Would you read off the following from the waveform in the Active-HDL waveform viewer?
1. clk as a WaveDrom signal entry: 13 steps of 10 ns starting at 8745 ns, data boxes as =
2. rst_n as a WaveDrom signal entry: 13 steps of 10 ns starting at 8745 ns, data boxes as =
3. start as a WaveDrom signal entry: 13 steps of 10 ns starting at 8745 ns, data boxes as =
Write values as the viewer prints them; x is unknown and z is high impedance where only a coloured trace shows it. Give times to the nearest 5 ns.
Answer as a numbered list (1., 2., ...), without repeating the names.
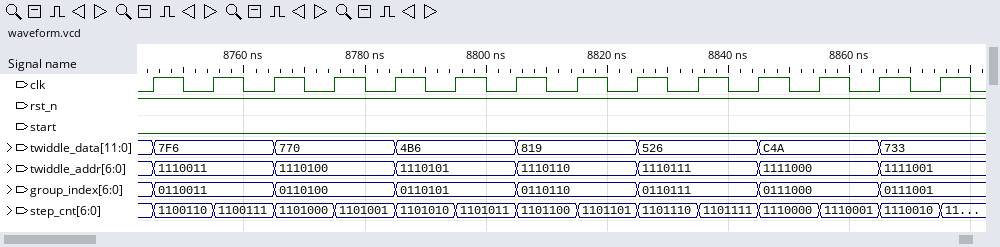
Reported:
1. {name: 'clk', wave: 'p............'}
2. {name: 'rst_n', wave: '1............'}
3. {name: 'start', wave: '0............'}
